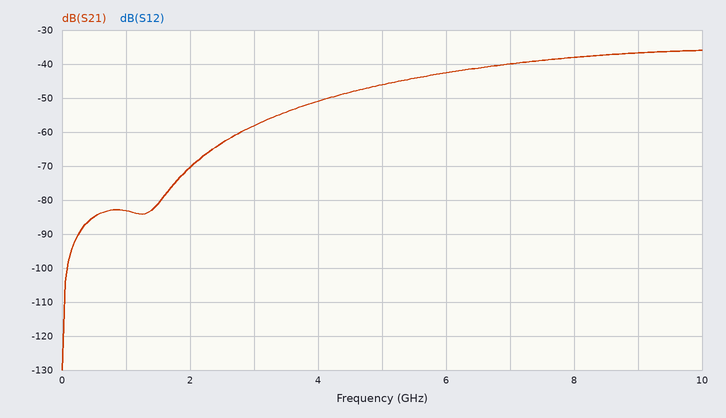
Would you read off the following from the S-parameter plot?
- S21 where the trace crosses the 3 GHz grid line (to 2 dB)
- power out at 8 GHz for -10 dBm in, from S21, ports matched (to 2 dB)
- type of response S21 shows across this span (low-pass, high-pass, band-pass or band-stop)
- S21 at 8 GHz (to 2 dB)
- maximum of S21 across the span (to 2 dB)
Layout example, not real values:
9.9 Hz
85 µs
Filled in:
-58 dB
-48 dBm
high-pass
-38 dB
-36 dB
